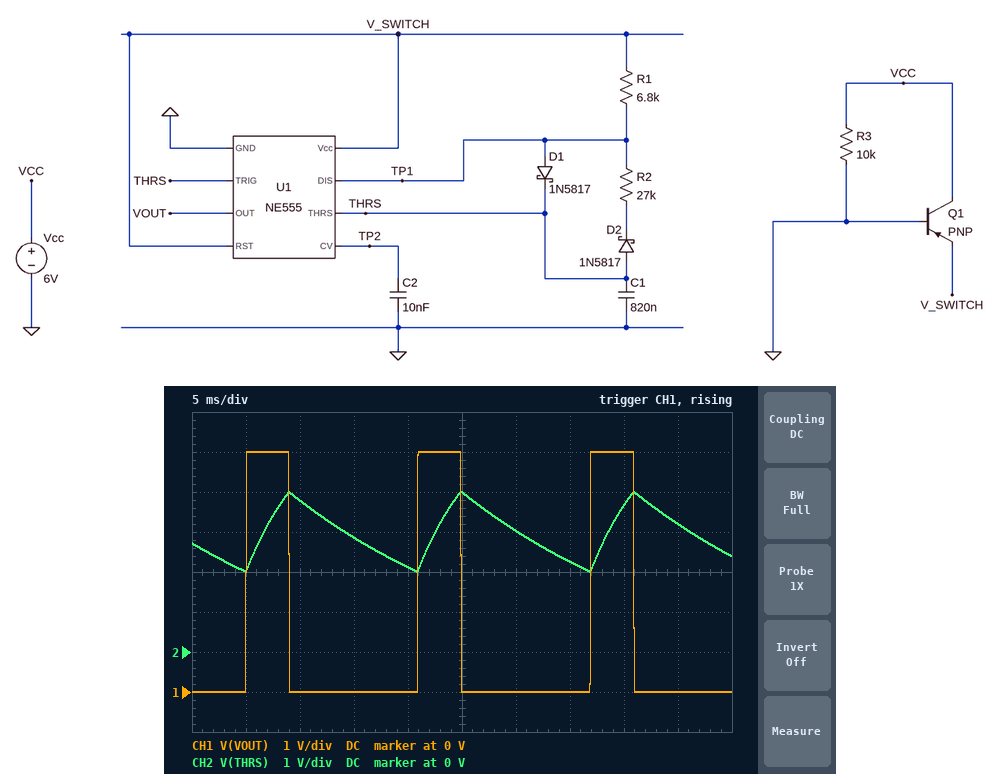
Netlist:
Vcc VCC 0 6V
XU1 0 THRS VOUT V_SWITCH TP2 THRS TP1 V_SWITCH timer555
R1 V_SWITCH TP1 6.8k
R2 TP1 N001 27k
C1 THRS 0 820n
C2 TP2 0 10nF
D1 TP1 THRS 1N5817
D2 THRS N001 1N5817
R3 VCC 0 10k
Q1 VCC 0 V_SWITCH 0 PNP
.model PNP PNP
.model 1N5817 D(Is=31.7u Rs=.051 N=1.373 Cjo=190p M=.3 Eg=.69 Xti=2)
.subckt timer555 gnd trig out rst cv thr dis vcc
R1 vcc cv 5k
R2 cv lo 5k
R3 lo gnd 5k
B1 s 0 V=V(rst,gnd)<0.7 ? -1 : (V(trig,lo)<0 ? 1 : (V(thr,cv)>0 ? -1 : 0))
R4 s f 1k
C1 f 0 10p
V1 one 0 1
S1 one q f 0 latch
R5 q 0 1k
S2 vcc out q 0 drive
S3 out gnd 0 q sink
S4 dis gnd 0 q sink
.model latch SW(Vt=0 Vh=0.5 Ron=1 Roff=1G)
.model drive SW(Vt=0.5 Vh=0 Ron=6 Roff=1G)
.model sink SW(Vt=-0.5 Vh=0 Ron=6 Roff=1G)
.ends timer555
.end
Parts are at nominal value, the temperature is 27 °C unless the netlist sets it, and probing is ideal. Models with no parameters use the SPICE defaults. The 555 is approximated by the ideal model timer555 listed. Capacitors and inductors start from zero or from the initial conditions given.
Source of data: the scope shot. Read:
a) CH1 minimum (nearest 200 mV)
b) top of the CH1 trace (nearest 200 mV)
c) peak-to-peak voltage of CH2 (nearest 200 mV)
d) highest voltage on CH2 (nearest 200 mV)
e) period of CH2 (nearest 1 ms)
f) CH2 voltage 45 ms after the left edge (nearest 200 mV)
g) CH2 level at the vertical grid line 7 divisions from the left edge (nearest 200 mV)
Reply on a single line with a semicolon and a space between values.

0 V; 6.0 V; 2.0 V; 4.0 V; 16 ms; 3.2 V; 2.2 V
